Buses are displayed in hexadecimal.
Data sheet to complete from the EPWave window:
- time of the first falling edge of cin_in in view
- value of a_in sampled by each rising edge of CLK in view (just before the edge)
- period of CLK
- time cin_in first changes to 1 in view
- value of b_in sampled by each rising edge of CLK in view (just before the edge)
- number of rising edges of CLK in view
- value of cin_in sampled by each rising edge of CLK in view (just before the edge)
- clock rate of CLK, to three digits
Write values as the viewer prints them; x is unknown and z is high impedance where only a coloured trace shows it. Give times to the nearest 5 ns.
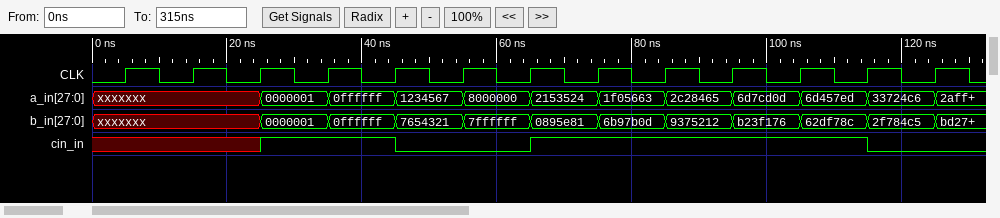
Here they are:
45 ns
xxxxxxx, xxxxxxx, xxxxxxx, 0000001, 0ffffff, 1234567, 8000000, 2153524, 1f05663, 2c28465, 6d7cd0d, 6d457ed, 33724c6
10 ns
25 ns
xxxxxxx, xxxxxxx, xxxxxxx, 0000001, 0ffffff, 7654321, 7ffffff, 0895e81, 6b97b0d, 9375212, b23f176, 62df78c, 2f784c5
13
x x x 1 1 0 0 1 1 1 1 1 0
100 MHz
